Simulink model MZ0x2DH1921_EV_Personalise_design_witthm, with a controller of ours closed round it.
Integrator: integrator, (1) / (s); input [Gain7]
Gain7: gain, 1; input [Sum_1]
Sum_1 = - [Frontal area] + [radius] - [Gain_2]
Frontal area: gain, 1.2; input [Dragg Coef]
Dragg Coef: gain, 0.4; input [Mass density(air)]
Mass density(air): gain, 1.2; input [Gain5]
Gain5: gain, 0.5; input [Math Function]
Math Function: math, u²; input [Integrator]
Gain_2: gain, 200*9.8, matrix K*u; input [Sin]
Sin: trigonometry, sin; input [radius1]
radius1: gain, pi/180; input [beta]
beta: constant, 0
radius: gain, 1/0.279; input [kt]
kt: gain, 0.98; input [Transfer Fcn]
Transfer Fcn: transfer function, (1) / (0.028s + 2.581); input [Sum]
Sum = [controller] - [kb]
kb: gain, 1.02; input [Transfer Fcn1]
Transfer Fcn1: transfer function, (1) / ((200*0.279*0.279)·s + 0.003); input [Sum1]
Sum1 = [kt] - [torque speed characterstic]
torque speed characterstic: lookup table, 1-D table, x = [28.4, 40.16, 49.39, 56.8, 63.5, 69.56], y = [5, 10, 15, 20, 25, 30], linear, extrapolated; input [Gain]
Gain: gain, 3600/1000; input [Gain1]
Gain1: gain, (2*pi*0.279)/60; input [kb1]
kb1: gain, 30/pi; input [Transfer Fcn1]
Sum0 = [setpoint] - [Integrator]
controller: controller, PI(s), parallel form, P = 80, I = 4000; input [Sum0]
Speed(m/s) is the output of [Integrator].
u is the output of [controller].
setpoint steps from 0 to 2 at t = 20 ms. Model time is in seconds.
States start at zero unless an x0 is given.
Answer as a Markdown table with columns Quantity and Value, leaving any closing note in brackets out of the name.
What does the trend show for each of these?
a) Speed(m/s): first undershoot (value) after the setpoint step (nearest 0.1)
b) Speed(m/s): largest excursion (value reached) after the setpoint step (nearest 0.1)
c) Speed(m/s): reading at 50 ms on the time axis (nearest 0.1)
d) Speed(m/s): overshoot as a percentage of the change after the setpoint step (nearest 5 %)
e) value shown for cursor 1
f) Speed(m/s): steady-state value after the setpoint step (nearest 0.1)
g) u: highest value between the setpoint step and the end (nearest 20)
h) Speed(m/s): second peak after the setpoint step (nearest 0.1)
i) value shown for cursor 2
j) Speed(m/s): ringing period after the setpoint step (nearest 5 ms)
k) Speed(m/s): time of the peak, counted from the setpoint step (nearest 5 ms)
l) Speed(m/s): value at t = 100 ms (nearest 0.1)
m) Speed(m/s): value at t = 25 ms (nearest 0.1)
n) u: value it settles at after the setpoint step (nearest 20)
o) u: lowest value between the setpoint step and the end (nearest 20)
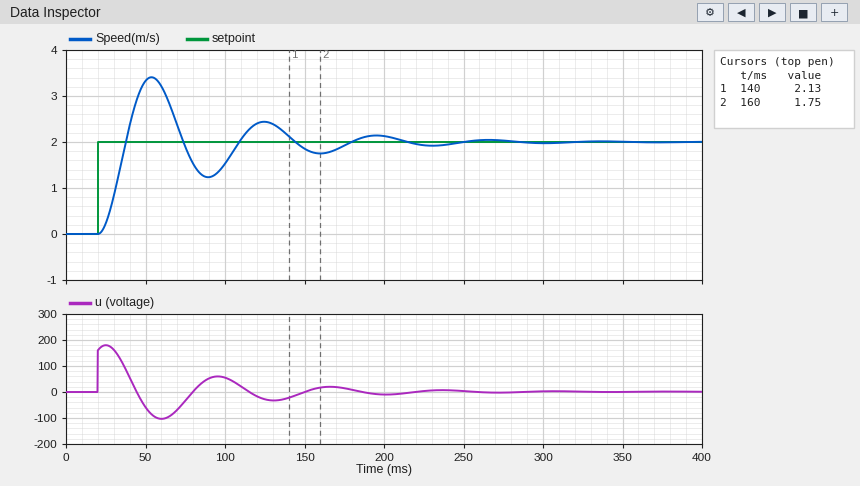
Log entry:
| Quantity | Value |
|---|---|
| Speed(m/s): first undershoot (value) after the setpoint step | 1.2 |
| Speed(m/s): largest excursion (value reached) after the setpoint step | 3.4 |
| Speed(m/s): reading at 50 ms on the time axis | 3.3 |
| Speed(m/s): overshoot as a percentage of the change after the setpoint step | 70 % |
| value shown for cursor 1 | 2.13 |
| Speed(m/s): steady-state value after the setpoint step | 2.0 |
| u: highest value between the setpoint step and the end | 180 |
| Speed(m/s): second peak after the setpoint step | 2.4 |
| value shown for cursor 2 | 1.75 |
| Speed(m/s): ringing period after the setpoint step | 70 ms |
| Speed(m/s): time of the peak, counted from the setpoint step | 35 ms |
| Speed(m/s): value at t = 100 ms | 1.5 |
| Speed(m/s): value at t = 25 ms | 0.2 |
| u: value it settles at after the setpoint step | 0 |
| u: lowest value between the setpoint step and the end | -100 |
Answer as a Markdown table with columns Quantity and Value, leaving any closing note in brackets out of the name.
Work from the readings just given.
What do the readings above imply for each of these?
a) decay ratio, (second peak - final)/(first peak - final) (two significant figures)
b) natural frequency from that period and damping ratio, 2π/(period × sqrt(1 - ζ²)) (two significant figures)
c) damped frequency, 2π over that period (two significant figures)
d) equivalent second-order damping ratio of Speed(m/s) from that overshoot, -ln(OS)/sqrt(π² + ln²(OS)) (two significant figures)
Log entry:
| Quantity | Value |
|---|---|
| decay ratio, (second peak - final)/(first peak - final) | 0.29 |
| natural frequency from that period and damping ratio, 2π/(period × sqrt(1 - ζ²)) | 0.090 rad/ms |
| damped frequency, 2π over that period | 0.090 rad/ms |
| equivalent second-order damping ratio of Speed(m/s) from that overshoot, -ln(OS)/sqrt(π² + ln²(OS)) | 0.11 |
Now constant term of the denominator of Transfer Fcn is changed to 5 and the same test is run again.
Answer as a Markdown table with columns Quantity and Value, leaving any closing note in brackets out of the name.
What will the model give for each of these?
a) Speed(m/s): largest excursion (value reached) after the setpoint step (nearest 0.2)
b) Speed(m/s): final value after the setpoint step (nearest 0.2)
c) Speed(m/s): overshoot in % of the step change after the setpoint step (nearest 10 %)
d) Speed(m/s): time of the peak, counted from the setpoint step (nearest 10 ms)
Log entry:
| Quantity | Value |
|---|---|
| Speed(m/s): largest excursion (value reached) after the setpoint step | 3.0 |
| Speed(m/s): final value after the setpoint step | 2.0 |
| Speed(m/s): overshoot in % of the step change after the setpoint step | 50 % |
| Speed(m/s): time of the peak, counted from the setpoint step | 40 ms |
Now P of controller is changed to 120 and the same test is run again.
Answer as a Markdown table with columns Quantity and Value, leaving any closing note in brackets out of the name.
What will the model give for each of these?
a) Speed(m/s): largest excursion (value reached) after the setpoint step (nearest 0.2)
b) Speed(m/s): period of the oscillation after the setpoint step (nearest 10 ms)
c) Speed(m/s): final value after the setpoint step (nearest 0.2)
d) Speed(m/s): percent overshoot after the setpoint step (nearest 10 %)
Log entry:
| Quantity | Value |
|---|---|
| Speed(m/s): largest excursion (value reached) after the setpoint step | 3.2 |
| Speed(m/s): period of the oscillation after the setpoint step | 60 ms |
| Speed(m/s): final value after the setpoint step | 2.0 |
| Speed(m/s): percent overshoot after the setpoint step | 60 % |
